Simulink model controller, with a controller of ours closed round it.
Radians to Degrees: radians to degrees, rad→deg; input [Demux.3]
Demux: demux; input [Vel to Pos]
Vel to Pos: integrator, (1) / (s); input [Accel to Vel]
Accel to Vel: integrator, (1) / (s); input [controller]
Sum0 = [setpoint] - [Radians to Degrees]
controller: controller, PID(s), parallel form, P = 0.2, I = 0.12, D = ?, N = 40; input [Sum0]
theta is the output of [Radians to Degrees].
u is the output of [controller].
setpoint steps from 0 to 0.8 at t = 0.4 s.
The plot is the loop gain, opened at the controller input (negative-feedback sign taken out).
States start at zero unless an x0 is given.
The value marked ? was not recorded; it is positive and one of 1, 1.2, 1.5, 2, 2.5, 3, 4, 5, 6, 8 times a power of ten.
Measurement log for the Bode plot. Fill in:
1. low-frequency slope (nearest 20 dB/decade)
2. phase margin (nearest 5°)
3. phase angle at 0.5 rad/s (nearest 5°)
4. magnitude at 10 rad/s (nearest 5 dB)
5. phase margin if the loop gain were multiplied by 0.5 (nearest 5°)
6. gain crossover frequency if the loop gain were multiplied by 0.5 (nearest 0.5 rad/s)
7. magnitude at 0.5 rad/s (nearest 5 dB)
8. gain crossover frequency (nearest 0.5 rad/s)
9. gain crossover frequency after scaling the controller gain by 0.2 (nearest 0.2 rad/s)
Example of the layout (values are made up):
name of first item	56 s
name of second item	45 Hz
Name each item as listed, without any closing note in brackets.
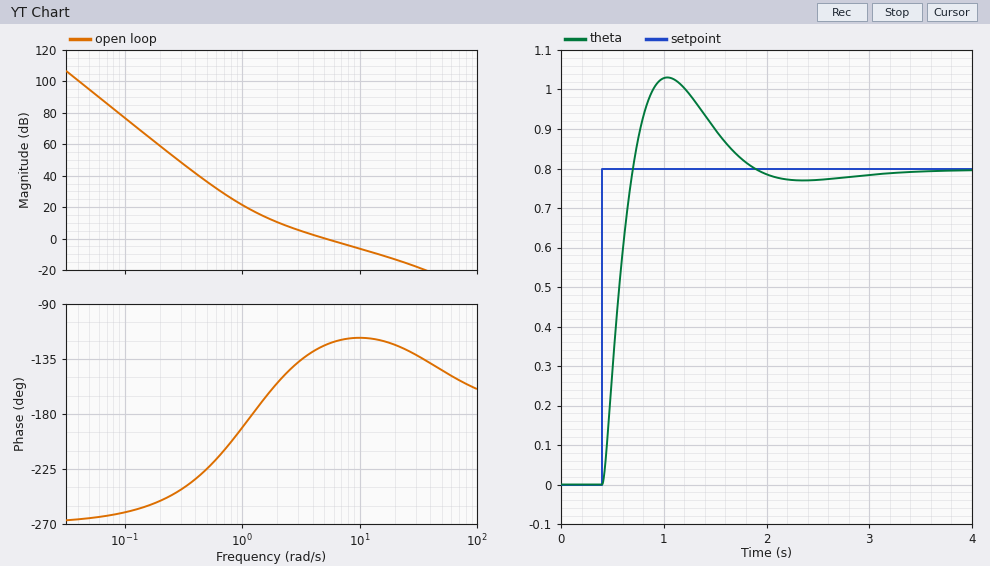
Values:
low-frequency slope	-60 dB/decade
phase margin	55°
phase angle at 0.5 rad/s	-225°
magnitude at 10 rad/s	-5 dB
phase margin if the loop gain were multiplied by 0.5	40°
gain crossover frequency if the loop gain were multiplied by 0.5	3.0 rad/s
magnitude at 0.5 rad/s	35 dB
gain crossover frequency	5.0 rad/s
gain crossover frequency after scaling the controller gain by 0.2	1.6 rad/s
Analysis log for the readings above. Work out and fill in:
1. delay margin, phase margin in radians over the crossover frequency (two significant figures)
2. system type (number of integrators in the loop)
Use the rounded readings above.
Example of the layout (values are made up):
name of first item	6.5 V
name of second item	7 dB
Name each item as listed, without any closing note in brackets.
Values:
delay margin, phase margin in radians over the crossover frequency	0.19 s
system type	3
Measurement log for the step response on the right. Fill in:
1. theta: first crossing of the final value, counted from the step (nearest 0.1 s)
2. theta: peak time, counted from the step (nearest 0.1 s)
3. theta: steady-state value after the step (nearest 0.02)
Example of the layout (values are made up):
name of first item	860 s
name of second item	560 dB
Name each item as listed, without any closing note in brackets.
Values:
theta: first crossing of the final value, counted from the step	0.3 s
theta: peak time, counted from the step	0.6 s
theta: steady-state value after the step	0.80
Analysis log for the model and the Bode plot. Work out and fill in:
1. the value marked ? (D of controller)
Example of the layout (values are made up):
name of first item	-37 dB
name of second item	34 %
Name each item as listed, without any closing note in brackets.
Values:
the value marked ?	0.08
